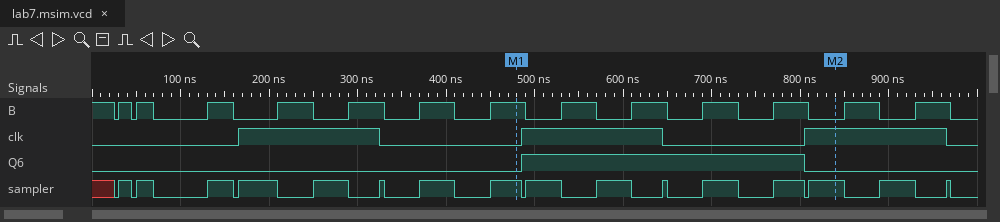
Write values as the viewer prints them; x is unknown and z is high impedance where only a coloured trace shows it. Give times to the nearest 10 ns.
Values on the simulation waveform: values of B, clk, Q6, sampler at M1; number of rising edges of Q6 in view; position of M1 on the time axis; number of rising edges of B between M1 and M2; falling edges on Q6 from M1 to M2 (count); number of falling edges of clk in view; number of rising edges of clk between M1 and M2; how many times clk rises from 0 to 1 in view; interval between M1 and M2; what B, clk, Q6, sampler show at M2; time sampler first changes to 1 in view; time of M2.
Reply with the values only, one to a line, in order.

B=1, clk=0, Q6=0, sampler=1
1
480 ns
4
1
3
2
3
360 ns
B=0, clk=1, Q6=0, sampler=1
30 ns
840 ns
